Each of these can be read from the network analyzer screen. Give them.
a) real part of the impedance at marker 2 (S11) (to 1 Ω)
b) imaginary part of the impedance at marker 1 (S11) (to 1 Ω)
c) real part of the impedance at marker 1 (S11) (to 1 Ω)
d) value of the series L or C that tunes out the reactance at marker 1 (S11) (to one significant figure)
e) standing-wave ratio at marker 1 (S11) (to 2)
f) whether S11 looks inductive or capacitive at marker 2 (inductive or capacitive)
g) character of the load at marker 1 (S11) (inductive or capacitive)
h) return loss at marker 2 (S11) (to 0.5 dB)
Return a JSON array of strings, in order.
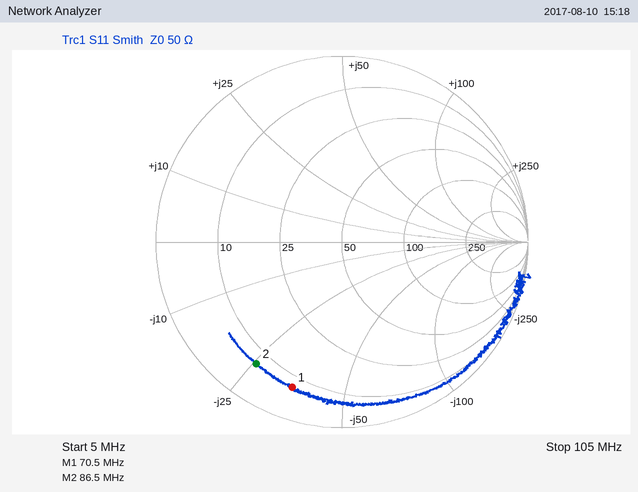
["7 Ω", "-35 Ω", "7 Ω", "80 nH", "10", "capacitive", "capacitive", "2.0 dB"]
